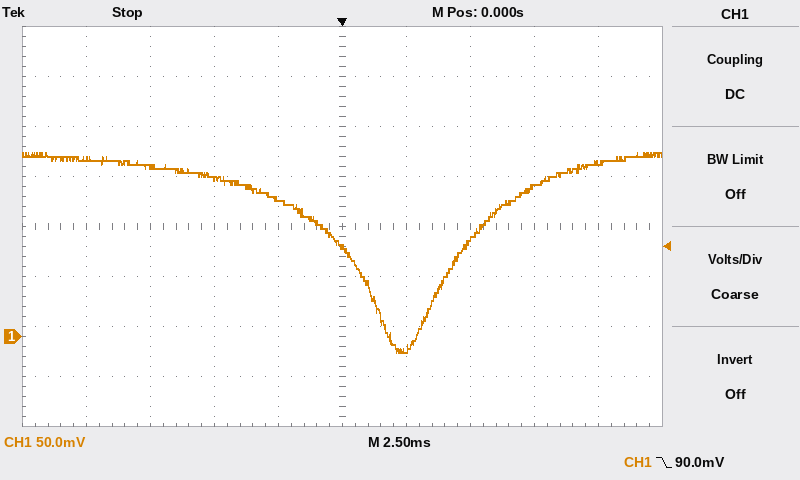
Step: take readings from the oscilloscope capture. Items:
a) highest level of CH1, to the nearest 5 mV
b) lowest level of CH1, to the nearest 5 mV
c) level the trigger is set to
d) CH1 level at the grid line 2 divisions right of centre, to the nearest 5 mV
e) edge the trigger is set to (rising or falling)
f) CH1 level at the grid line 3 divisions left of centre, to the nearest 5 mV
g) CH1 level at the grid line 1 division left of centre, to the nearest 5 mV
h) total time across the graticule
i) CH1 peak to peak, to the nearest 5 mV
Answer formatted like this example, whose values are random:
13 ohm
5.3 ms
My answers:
185 mV
-15 mV
90.0 mV
95 mV
falling
170 mV
140 mV
25 ms
200 mV
